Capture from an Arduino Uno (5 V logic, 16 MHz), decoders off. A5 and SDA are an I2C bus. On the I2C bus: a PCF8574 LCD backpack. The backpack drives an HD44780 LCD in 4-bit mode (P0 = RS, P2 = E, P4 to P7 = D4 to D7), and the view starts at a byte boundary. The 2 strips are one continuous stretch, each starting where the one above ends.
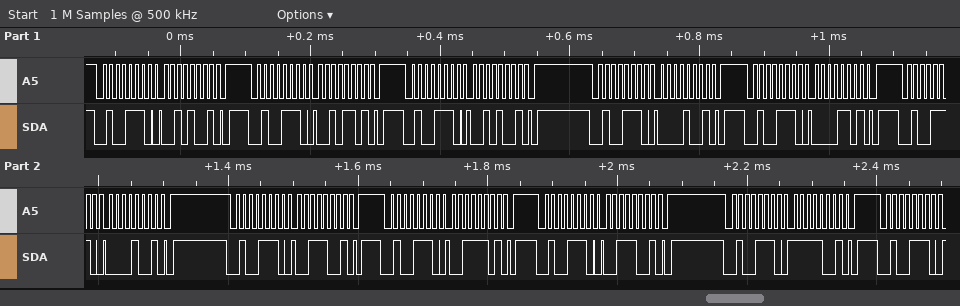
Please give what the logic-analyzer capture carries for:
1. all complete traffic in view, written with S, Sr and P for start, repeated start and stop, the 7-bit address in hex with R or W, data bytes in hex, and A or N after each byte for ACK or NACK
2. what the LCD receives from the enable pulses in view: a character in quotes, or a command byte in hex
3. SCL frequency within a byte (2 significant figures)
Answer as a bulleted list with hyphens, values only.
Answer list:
- S 27W A 29 A P S 27W A 2D A P S 27W A 29 A P S 27W A 09 A P S 27W A 0D A P S 27W A 09 A P S 27W A 39 A P S 27W A 3D A P S 27W A 39 A P S 27W A F9 A P S 27W A
- ' '
- 100 kHz
